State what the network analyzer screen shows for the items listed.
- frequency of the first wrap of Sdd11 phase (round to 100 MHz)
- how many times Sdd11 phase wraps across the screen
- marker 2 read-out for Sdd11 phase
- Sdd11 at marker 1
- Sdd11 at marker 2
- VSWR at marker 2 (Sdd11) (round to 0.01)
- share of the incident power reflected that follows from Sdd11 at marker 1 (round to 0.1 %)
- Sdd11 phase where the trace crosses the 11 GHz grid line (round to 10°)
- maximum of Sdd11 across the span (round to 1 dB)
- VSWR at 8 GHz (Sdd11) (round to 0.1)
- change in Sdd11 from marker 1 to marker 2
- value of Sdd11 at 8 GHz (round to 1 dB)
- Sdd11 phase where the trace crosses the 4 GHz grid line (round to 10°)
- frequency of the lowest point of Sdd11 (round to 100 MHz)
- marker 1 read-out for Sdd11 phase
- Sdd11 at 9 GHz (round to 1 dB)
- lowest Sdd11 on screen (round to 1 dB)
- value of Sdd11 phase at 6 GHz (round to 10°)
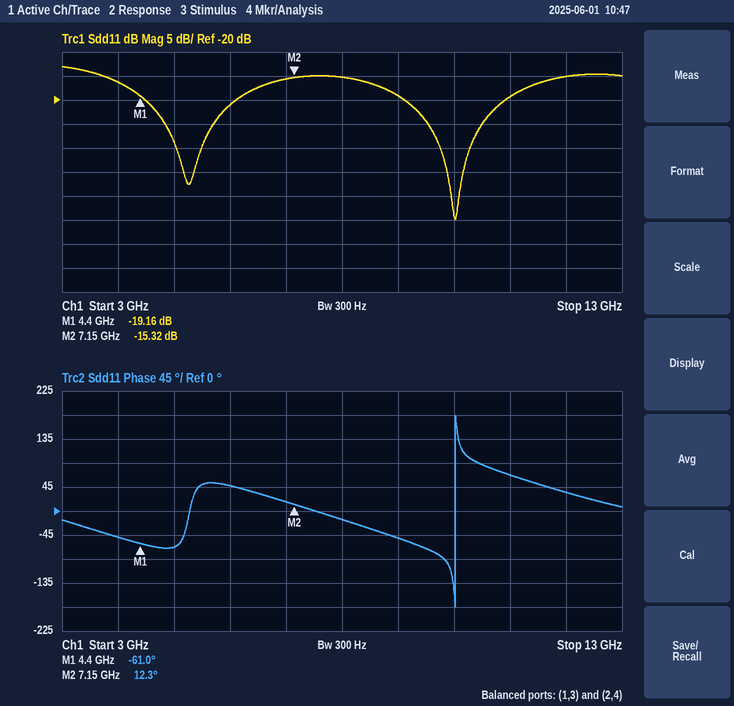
10.0 GHz
1
12.3°
-19.16 dB
-15.32 dB
1.41
1.2 %
70°
-13 dB
1.4
3.84 dB
-15 dB
-50°
10.0 GHz
-61.0°
-19 dB
-45 dB
50°
